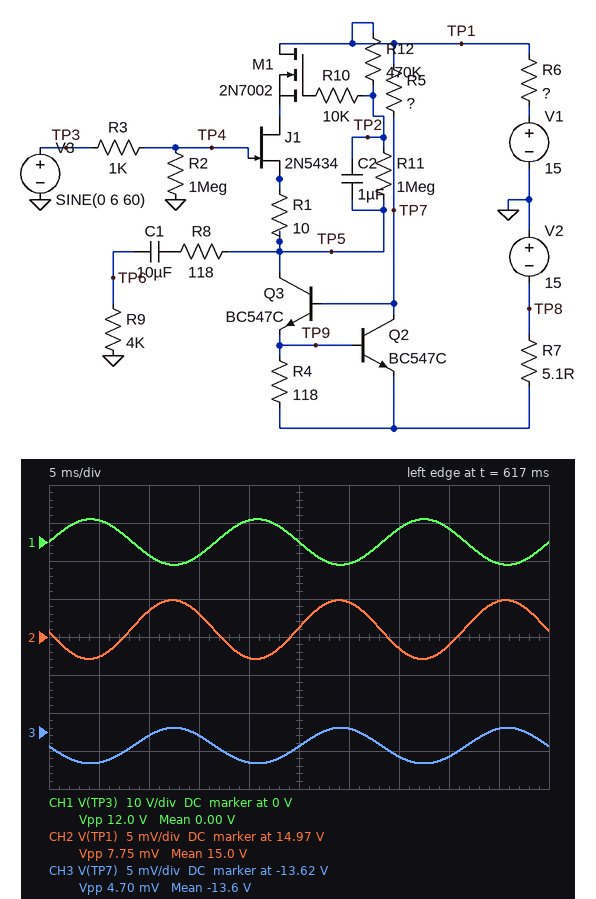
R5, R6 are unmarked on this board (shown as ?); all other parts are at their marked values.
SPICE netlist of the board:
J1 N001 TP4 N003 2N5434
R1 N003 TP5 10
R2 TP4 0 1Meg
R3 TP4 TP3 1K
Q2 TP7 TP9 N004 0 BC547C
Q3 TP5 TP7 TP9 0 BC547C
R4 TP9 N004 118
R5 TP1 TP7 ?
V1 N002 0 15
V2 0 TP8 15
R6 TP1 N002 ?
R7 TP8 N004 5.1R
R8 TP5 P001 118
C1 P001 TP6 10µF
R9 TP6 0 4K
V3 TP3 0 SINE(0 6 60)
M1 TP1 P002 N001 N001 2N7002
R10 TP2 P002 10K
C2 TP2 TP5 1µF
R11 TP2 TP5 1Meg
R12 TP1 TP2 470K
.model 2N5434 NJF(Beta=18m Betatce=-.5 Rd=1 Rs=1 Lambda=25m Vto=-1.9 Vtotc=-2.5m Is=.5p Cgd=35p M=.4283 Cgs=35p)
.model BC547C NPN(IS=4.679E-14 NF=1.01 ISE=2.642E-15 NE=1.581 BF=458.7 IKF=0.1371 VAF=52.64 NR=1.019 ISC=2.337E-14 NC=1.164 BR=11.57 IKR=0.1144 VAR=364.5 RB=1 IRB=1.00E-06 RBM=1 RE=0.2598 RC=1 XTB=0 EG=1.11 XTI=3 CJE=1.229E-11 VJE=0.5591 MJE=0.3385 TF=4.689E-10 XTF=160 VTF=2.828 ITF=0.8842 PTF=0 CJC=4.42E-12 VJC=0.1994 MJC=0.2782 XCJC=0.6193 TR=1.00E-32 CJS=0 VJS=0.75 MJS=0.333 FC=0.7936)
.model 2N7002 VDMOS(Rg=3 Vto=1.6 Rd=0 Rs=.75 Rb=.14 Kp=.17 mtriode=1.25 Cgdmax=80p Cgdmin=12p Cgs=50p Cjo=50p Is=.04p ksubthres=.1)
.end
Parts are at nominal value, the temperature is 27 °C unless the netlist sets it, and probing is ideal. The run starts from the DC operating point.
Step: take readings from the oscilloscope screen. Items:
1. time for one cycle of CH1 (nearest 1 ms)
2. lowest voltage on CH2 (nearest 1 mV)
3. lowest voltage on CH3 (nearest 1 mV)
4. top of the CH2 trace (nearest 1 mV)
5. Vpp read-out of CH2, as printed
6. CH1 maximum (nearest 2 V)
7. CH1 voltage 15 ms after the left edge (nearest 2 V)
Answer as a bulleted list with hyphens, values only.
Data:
- 17 ms
- 14.967 V
- -13.619 V
- 14.975 V
- 7.75 mV
- 6 V
- -4 V
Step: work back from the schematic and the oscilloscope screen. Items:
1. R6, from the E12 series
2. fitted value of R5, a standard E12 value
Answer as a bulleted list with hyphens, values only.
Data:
- 2.7 Ω
- 5.6 kΩ
